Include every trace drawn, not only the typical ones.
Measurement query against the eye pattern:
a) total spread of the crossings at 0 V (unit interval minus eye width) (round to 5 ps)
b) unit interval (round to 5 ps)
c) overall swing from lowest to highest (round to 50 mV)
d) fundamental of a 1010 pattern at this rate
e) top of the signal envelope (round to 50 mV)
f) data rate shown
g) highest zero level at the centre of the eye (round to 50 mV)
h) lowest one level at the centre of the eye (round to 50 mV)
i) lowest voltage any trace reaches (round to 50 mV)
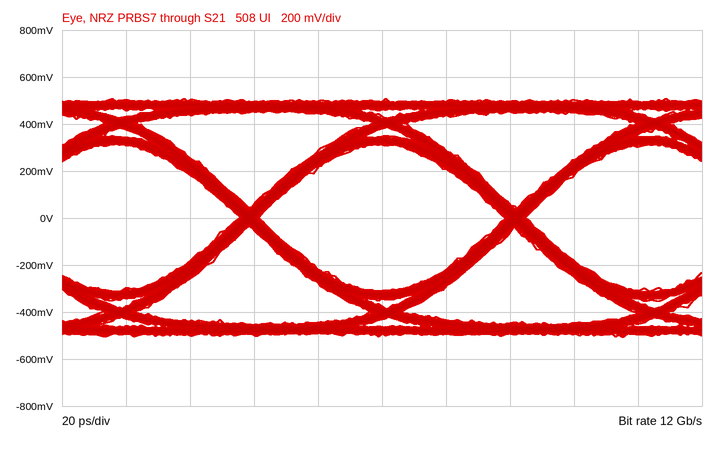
5 ps
85 ps
1.00 V
6 GHz
500 mV
12 Gb/s
-300 mV
300 mV
-500 mV
